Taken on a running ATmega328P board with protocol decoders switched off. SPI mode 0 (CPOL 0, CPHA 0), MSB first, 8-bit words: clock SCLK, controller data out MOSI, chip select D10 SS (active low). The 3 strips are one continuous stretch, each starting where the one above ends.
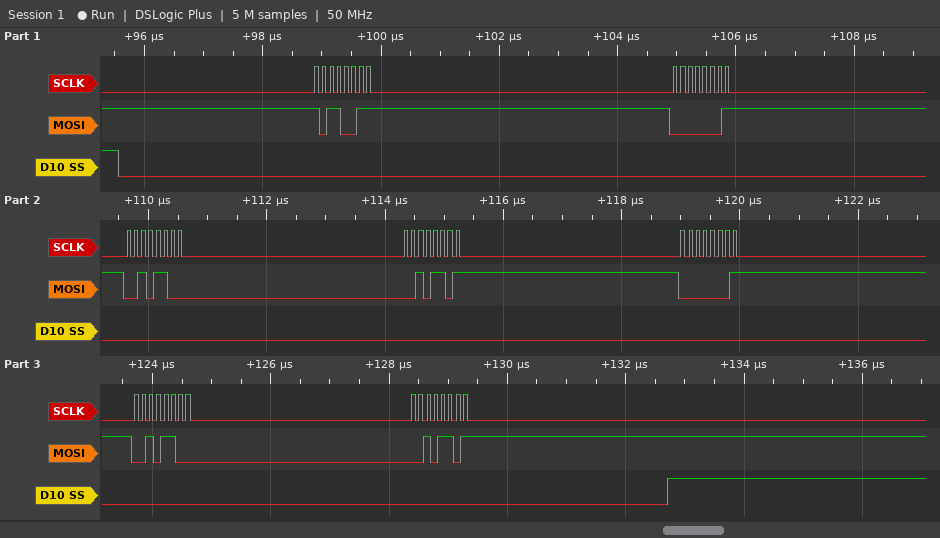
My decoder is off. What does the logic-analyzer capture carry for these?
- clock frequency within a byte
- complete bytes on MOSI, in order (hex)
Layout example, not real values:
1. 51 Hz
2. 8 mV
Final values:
1. 8 MHz
2. B3 01 2C 2D 01 2C 2D
